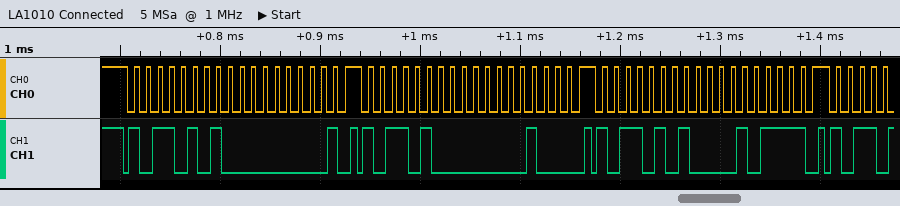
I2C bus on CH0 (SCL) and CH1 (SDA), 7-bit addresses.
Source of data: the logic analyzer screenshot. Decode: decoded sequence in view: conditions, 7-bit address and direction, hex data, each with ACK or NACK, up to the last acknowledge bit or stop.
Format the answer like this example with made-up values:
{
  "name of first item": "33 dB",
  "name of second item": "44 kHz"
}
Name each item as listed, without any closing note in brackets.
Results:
{
  "decoded sequence in view: conditions, 7-bit address and direction, hex data, each with ACK or NACK, up to the last acknowledge bit or stop": "start, address 5A read ACK, 00 NACK, stop, start, address 5A write ACK, 04 ACK, stop, start, address 5A read ACK, 17 NACK, stop"
}
